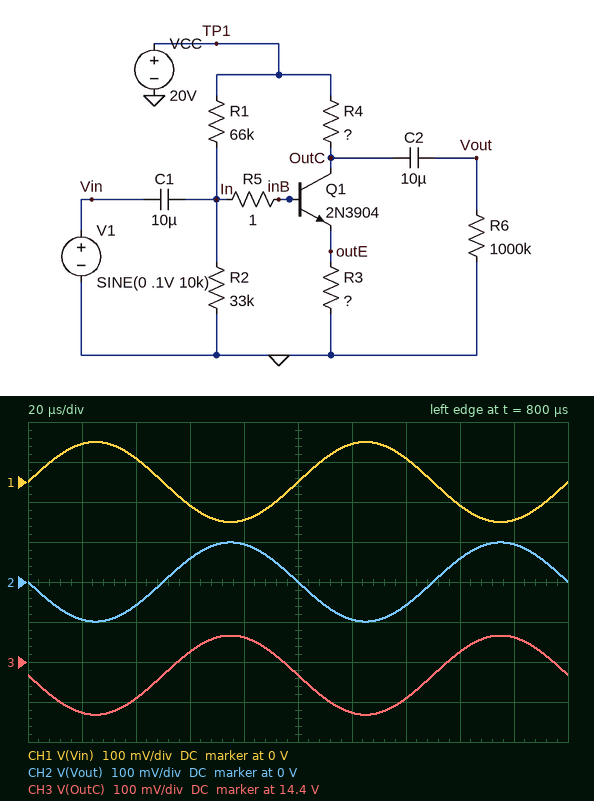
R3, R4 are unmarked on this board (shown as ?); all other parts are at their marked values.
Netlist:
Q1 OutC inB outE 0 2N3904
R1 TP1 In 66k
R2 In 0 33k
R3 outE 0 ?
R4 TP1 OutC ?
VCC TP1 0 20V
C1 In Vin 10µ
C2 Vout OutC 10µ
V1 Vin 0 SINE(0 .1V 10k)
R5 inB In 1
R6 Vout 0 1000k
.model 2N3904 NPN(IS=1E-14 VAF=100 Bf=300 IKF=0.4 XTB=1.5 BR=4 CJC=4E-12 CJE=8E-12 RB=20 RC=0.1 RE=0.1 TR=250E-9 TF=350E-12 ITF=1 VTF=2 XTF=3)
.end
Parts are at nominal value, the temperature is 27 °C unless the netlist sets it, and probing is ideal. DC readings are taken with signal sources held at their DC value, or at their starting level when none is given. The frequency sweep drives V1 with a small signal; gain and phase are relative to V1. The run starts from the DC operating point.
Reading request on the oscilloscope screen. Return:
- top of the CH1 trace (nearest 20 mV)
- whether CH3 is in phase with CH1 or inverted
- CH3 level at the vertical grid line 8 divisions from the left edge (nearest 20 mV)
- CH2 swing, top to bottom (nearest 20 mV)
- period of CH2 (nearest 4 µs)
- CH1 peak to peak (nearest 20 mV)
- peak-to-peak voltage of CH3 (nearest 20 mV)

100 mV
inverted
14.42 V
200 mV
100 µs
200 mV
200 mV
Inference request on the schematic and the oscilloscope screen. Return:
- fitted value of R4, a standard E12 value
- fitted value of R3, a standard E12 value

1.2 kΩ
1.2 kΩ
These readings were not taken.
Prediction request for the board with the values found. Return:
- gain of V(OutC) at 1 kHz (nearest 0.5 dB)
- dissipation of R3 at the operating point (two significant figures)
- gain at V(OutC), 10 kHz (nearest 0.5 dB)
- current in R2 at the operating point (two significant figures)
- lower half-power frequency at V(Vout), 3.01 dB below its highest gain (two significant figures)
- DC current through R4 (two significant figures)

0 dB
27 mW
0 dB
190 µA
930 mHz
4.7 mA
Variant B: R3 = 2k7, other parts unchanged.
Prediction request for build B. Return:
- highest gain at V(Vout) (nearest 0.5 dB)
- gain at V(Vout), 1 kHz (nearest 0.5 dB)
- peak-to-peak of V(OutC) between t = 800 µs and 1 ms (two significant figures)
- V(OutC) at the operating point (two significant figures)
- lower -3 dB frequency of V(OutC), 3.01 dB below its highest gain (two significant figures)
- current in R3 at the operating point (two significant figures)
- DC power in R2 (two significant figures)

0 dB
-7.0 dB
88 mV
17 V
55 MHz
2.2 mA
1.3 mW
